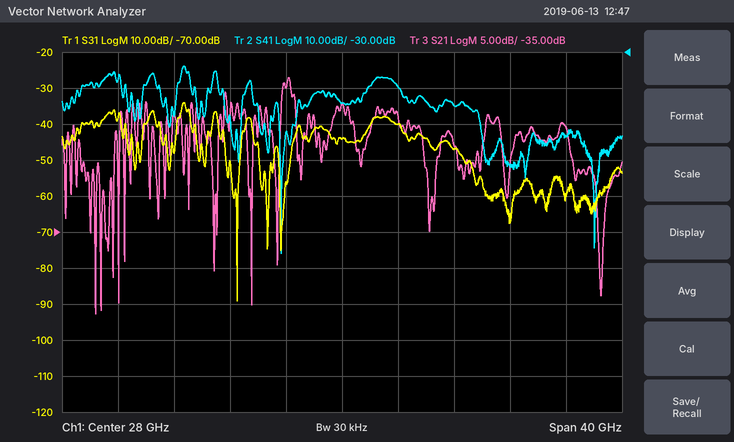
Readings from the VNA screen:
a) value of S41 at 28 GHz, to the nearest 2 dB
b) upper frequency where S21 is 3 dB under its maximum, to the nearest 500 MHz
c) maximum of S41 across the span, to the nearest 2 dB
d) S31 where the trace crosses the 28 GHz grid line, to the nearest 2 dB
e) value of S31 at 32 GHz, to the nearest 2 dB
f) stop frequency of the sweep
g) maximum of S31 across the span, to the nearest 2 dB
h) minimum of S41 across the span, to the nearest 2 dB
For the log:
-44 dB
24.5 GHz
-34 dB
-44 dB
-40 dB
48 GHz
-34 dB
-86 dB
